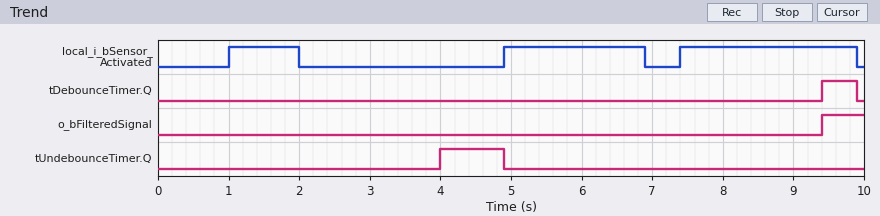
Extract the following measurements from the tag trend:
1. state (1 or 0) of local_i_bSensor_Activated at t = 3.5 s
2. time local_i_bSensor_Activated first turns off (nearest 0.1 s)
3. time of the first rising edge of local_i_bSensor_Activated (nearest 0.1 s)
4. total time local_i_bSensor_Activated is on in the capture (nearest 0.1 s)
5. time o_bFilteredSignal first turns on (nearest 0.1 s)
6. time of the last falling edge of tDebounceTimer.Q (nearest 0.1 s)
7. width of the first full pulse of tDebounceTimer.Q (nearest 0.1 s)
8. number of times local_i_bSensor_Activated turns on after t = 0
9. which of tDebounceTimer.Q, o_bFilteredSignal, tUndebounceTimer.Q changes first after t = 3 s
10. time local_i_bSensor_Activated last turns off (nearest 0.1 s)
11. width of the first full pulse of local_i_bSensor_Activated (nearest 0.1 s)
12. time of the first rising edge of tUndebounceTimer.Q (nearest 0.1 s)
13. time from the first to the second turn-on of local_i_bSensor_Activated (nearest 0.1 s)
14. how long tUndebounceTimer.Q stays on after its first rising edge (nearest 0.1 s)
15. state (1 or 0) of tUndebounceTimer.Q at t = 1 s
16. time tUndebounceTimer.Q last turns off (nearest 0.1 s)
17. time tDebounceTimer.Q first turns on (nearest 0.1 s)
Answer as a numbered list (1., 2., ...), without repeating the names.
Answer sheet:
1. 0
2. 2.0 s
3. 1.0 s
4. 5.5 s
5. 9.4 s
6. 9.9 s
7. 0.5 s
8. 3
9. tUndebounceTimer.Q
10. 9.9 s
11. 1.0 s
12. 4.0 s
13. 3.9 s
14. 0.9 s
15. 0
16. 4.9 s
17. 9.4 s
